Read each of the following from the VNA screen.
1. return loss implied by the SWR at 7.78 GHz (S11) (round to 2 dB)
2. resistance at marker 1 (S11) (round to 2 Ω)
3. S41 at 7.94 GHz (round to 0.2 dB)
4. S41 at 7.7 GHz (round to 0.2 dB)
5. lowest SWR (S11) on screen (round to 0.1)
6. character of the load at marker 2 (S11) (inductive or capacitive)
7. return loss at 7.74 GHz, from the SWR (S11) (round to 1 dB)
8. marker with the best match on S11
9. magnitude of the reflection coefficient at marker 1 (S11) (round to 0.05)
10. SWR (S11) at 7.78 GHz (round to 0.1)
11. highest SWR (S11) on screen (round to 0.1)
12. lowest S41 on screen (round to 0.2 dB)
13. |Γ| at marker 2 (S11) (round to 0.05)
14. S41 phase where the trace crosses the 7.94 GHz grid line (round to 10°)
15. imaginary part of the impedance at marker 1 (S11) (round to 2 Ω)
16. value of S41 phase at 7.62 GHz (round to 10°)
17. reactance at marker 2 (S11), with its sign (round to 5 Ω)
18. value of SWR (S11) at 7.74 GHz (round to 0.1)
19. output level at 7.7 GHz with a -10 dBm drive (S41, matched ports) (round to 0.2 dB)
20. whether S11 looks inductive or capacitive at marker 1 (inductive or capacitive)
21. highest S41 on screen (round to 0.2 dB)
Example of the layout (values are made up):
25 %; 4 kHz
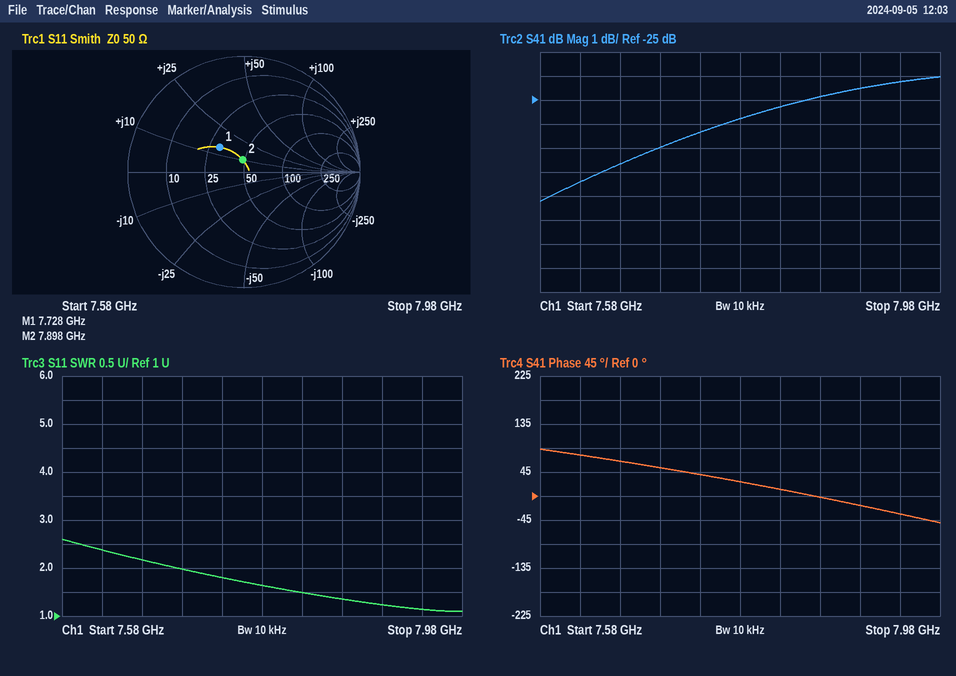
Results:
12 dB; 30 Ω; -24.2 dB; -27.0 dB; 1.1; inductive; 11 dB; marker 2; 0.30; 1.6; 2.6; -29.2 dB; 0.10; -30°; +14 Ω; 80°; +10 Ω; 1.8; -37.0 dBm; inductive; -24.0 dB
